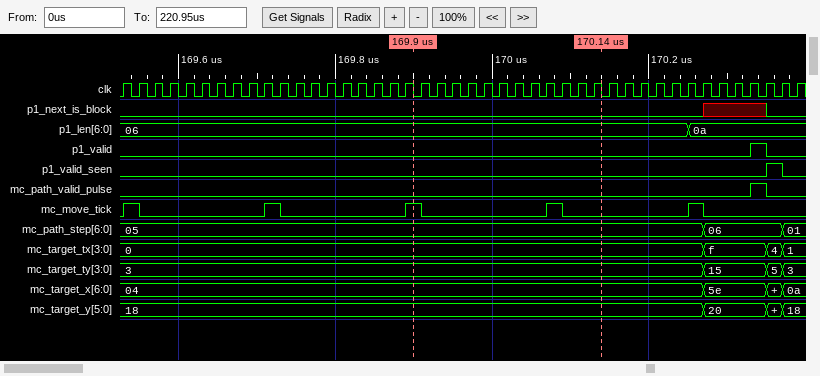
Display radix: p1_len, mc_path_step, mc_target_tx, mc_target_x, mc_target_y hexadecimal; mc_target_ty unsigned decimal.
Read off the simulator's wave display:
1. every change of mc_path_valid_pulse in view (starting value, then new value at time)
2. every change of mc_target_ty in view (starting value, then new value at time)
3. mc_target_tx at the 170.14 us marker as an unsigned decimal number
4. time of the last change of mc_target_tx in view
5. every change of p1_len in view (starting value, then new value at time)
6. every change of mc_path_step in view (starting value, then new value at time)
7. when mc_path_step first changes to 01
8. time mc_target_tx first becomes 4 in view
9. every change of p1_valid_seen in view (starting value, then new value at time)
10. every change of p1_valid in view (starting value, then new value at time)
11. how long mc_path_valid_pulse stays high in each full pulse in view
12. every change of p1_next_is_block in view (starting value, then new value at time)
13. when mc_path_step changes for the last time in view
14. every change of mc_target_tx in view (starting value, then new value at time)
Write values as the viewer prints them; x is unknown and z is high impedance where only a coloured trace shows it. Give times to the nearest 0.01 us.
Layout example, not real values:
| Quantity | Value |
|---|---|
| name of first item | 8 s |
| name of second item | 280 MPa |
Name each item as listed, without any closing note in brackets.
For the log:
| Quantity | Value |
|---|---|
| every change of mc_path_valid_pulse in view | 0, 1 at 170.33 us, 0 at 170.35 us |
| every change of mc_target_ty in view | 3, 15 at 170.27 us, 5 at 170.35 us, 3 at 170.37 us |
| mc_target_tx at the 170.14 us marker as an unsigned decimal number | 0 |
| time of the last change of mc_target_tx in view | 170.37 us |
| every change of p1_len in view | 06, 0a at 170.25 us |
| every change of mc_path_step in view | 05, 06 at 170.27 us, 01 at 170.37 us |
| when mc_path_step first changes to 01 | 170.37 us |
| time mc_target_tx first becomes 4 in view | 170.35 us |
| every change of p1_valid_seen in view | 0, 1 at 170.35 us, 0 at 170.37 us |
| every change of p1_valid in view | 0, 1 at 170.33 us, 0 at 170.35 us |
| how long mc_path_valid_pulse stays high in each full pulse in view | 0.02 us |
| every change of p1_next_is_block in view | 0, x at 170.27 us, 0 at 170.35 us |
| when mc_path_step changes for the last time in view | 170.37 us |
| every change of mc_target_tx in view | 0, f at 170.27 us, 4 at 170.35 us, 1 at 170.37 us |
